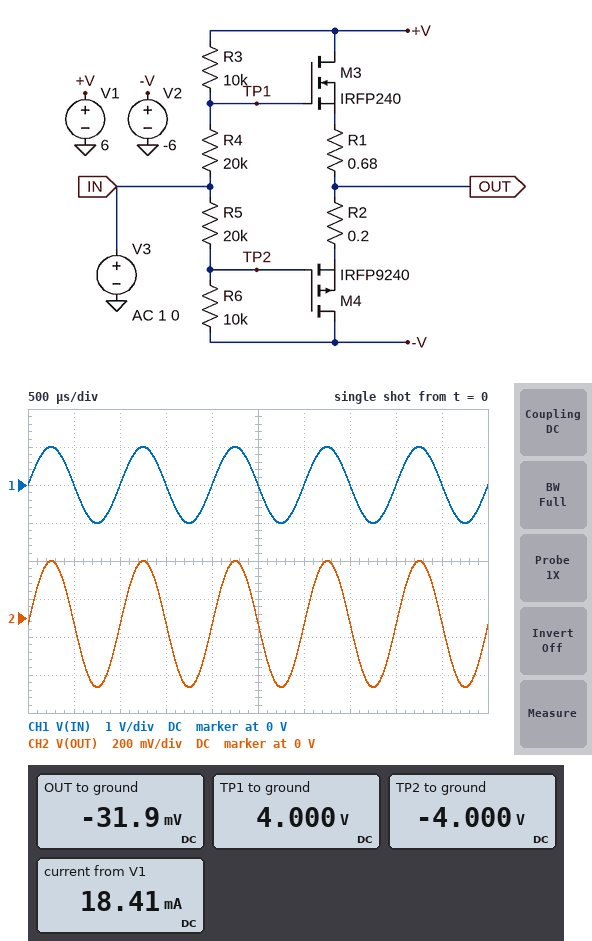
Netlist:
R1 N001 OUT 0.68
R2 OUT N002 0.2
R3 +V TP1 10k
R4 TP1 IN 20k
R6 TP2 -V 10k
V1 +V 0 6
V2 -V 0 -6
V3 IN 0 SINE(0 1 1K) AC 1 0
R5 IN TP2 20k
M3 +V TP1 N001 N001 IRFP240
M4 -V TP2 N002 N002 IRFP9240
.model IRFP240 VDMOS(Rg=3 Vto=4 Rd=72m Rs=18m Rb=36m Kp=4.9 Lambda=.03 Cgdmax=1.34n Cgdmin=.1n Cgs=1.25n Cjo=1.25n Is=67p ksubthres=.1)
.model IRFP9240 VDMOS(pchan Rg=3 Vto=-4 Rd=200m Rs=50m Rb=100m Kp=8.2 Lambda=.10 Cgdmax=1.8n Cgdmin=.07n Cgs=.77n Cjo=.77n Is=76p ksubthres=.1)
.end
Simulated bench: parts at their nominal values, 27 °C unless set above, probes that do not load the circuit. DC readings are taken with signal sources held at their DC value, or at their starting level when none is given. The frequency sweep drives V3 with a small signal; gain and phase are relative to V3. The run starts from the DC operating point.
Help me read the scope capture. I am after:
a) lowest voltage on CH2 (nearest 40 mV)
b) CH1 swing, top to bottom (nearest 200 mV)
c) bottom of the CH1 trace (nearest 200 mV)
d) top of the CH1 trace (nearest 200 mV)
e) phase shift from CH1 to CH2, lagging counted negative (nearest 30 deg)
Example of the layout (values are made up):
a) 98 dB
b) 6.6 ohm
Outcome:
a) -360 mV
b) 2.0 V
c) -1.0 V
d) 1.0 V
e) 0 deg
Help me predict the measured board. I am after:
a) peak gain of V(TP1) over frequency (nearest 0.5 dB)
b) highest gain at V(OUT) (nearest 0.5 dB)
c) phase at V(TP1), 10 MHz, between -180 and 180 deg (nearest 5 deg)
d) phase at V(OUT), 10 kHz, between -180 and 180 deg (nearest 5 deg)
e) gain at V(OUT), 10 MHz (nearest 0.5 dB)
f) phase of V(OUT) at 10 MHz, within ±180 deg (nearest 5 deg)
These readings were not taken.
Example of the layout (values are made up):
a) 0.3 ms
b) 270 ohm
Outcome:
a) -9.5 dB
b) -9.5 dB
c) -95 deg
d) -10 deg
e) -54.0 dB
f) -105 deg
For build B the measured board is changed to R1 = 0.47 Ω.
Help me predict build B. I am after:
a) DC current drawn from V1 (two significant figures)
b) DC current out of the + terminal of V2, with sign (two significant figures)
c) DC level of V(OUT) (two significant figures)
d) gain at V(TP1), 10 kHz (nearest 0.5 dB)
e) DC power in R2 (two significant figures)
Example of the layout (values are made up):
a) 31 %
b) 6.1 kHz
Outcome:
a) 19 mA
b) -19 mA
c) -30 mV
d) -9.5 dB
e) 70 µW
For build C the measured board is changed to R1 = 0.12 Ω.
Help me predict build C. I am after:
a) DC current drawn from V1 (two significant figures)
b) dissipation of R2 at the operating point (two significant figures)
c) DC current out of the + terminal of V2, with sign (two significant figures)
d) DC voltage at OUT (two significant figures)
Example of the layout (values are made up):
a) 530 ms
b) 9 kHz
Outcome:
a) 20 mA
b) 76 µW
c) -20 mA
d) -27 mV
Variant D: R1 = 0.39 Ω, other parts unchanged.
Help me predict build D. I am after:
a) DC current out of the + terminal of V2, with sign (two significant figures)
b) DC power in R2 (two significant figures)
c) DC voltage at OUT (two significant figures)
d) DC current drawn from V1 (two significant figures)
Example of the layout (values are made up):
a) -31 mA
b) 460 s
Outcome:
a) -19 mA
b) 71 µW
c) -29 mV
d) 19 mA
